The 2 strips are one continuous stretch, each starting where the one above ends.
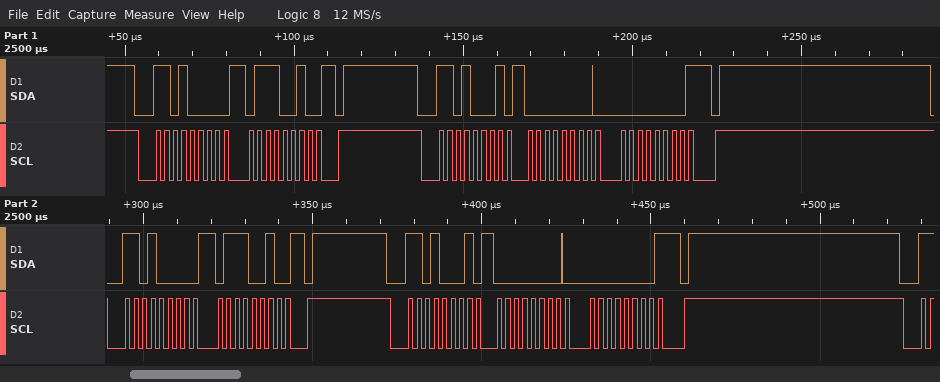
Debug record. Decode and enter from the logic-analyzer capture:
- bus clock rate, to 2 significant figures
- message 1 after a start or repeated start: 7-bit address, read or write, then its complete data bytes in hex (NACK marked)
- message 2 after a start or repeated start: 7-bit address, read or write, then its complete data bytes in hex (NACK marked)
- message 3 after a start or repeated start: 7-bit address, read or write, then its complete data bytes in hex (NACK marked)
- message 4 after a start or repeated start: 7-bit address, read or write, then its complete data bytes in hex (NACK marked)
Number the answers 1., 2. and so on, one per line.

1. 400 kHz
2. 0x68 write: 72
3. 0x68 read: 00 00 NACK
4. 0x68 write: 72
5. 0x68 read: 00 00 NACK
